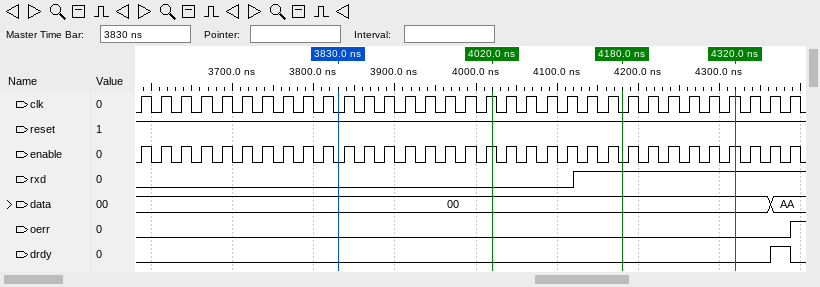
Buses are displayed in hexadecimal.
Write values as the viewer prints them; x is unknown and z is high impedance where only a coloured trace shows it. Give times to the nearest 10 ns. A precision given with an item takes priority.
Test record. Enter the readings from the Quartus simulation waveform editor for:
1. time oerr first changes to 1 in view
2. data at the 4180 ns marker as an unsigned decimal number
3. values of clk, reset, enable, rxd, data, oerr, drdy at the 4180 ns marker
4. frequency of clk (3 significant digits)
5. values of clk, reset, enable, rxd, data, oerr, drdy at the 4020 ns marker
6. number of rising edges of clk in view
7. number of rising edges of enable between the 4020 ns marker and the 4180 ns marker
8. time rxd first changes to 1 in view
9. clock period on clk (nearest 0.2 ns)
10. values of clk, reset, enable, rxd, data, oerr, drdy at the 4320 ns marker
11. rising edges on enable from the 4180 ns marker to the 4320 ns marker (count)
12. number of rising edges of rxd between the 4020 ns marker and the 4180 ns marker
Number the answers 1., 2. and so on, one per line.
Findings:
1. 4390 ns
2. 0
3. clk=0, reset=1, enable=0, rxd=1, data=00, oerr=0, drdy=0
4. 40.0 MHz
5. clk=1, reset=1, enable=1, rxd=0, data=00, oerr=0, drdy=0
6. 33
7. 6
8. 4120 ns
9. 25 ns
10. clk=1, reset=1, enable=1, rxd=1, data=00, oerr=0, drdy=0
11. 6
12. 1
